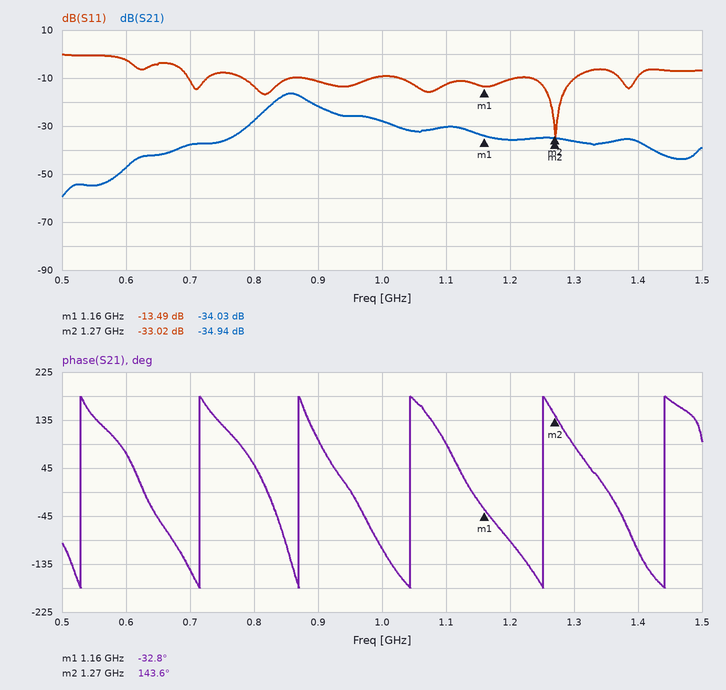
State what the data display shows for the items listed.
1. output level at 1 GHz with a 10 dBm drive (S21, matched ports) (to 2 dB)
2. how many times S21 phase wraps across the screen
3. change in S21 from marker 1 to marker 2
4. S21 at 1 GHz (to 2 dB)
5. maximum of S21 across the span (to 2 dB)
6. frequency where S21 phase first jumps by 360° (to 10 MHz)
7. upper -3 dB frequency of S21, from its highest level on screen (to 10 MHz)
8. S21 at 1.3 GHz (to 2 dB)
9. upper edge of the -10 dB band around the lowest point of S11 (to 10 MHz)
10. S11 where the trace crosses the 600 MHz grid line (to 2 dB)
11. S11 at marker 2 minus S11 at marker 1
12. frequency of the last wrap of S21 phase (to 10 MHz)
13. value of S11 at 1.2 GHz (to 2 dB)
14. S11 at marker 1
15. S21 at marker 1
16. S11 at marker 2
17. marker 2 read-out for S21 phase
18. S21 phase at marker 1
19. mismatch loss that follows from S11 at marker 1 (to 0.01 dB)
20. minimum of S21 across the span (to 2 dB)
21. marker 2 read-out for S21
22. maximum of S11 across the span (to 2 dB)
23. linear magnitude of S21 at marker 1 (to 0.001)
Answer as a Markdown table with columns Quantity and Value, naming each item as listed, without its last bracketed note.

| Quantity | Value |
|---|---|
| output level at 1 GHz with a 10 dBm drive (S21, matched ports) | -18 dBm |
| how many times S21 phase wraps across the screen | 6 |
| change in S21 from marker 1 to marker 2 | -0.91 dB |
| S21 at 1 GHz | -28 dB |
| maximum of S21 across the span | -16 dB |
| frequency where S21 phase first jumps by 360° | 530 MHz |
| upper -3 dB frequency of S21, from its highest level on screen | 880 MHz |
| S21 at 1.3 GHz | -36 dB |
| upper edge of the -10 dB band around the lowest point of S11 | 1.30 GHz |
| S11 where the trace crosses the 600 MHz grid line | -2 dB |
| S11 at marker 2 minus S11 at marker 1 | -19.53 dB |
| frequency of the last wrap of S21 phase | 1.44 GHz |
| value of S11 at 1.2 GHz | -10 dB |
| S11 at marker 1 | -13.49 dB |
| S21 at marker 1 | -34.03 dB |
| S11 at marker 2 | -33.02 dB |
| marker 2 read-out for S21 phase | 143.6° |
| S21 phase at marker 1 | -32.8° |
| mismatch loss that follows from S11 at marker 1 | 0.20 dB |
| minimum of S21 across the span | -60 dB |
| marker 2 read-out for S21 | -34.94 dB |
| maximum of S11 across the span | 0 dB |
| linear magnitude of S21 at marker 1 | 0.020 |
